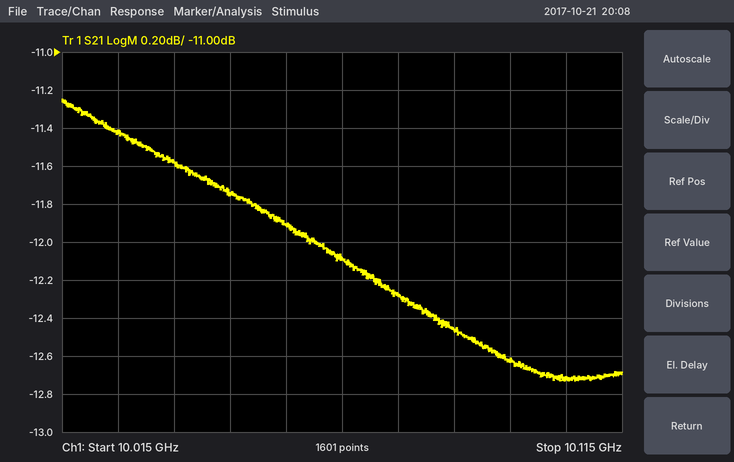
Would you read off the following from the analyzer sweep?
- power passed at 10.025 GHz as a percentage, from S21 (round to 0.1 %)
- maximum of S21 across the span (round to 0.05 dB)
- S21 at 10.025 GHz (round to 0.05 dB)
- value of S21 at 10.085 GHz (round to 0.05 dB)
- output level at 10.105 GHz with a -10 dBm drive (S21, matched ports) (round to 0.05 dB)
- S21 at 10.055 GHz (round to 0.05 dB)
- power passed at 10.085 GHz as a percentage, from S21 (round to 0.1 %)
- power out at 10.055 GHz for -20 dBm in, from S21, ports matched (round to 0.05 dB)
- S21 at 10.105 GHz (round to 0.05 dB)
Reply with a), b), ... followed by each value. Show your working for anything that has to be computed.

a) 10^(-11.4/10) ≈ 7.2 %
b) -11.25 dB
c) -11.40 dB
d) -12.45 dB
e) -10 dBm + (-12.70 dB) = -22.70 dBm
f) -11.90 dB
g) 10^(-12.45/10) ≈ 5.7 %
h) -20 dBm + (-11.90 dB) = -31.90 dBm
i) -12.70 dB
